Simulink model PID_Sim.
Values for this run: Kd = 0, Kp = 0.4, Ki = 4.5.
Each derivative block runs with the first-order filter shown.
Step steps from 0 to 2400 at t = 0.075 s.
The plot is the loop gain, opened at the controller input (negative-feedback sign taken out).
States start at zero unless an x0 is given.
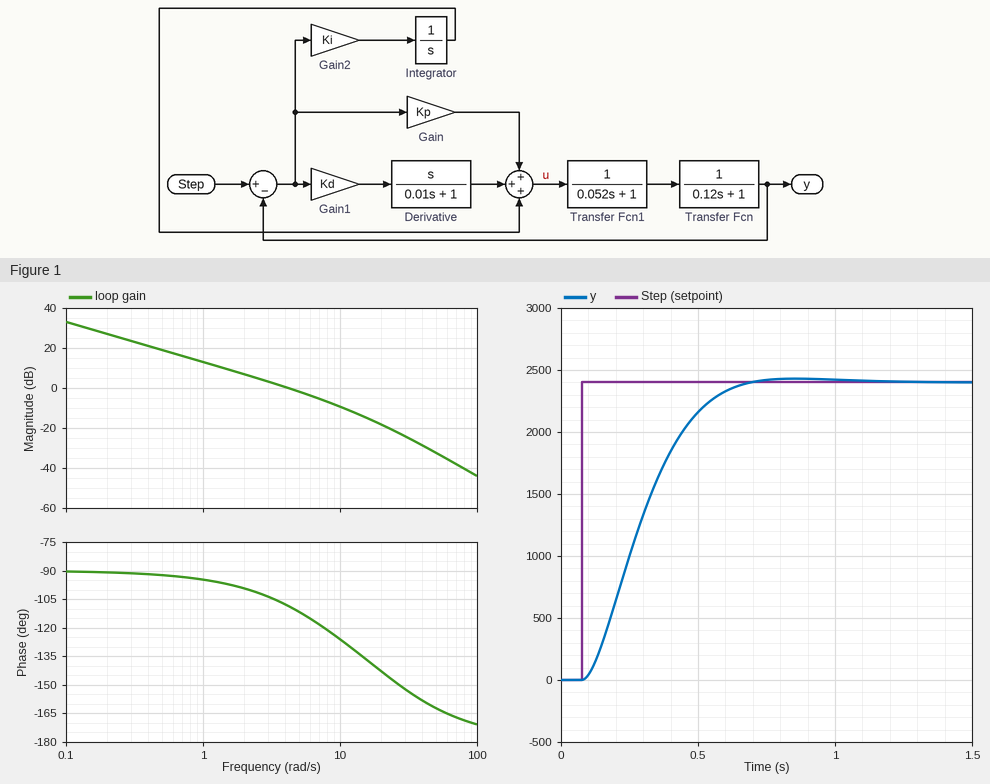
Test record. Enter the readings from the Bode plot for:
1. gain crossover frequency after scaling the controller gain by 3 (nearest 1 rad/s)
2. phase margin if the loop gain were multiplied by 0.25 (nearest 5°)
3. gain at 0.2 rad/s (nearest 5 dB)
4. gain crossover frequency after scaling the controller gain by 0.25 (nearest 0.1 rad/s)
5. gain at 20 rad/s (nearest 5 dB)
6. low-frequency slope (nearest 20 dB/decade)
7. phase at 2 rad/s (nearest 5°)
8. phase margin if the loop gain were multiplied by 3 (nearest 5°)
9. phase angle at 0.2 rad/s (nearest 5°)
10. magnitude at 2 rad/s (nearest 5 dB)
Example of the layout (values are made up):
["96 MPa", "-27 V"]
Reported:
["10 rad/s", "85°", "25 dB", "1.1 rad/s", "-20 dB", "-20 dB/decade", "-100°", "55°", "-90°", "5 dB"]
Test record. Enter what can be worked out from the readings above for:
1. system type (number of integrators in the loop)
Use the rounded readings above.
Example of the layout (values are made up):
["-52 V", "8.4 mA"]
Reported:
["1"]
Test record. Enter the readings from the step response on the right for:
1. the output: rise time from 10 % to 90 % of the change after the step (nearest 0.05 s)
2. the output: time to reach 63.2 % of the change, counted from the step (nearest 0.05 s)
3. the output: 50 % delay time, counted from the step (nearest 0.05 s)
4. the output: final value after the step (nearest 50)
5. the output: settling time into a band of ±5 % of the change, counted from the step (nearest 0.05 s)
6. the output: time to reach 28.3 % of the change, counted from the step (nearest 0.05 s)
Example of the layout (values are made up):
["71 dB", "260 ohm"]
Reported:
["0.35 s", "0.25 s", "0.20 s", "2400", "0.50 s", "0.15 s"]
